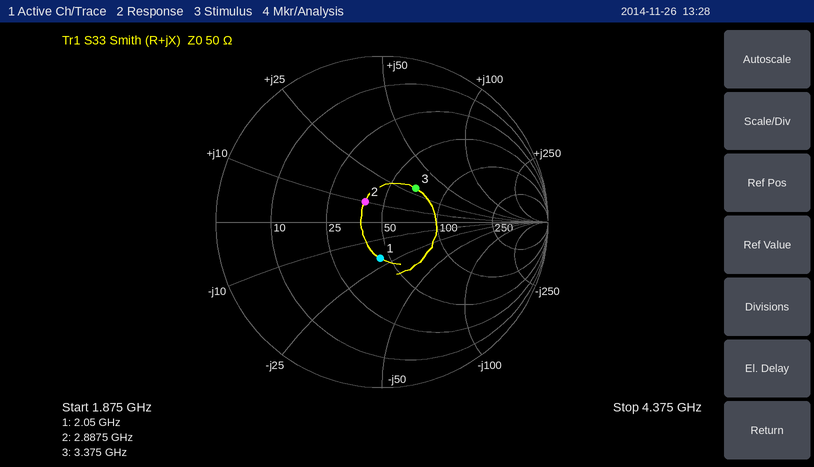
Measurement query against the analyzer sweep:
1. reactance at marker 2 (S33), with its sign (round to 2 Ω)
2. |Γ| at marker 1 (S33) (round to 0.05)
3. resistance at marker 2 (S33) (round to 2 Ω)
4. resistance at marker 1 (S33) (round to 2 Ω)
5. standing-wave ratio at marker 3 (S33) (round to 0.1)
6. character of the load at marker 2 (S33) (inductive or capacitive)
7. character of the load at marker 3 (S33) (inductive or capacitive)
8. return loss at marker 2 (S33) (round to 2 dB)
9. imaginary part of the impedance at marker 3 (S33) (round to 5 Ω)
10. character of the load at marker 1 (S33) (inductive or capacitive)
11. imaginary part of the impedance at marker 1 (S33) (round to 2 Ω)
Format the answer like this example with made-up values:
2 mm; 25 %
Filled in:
+10 Ω; 0.20; 40 Ω; 44 Ω; 1.8; inductive; inductive; 16 dB; +30 Ω; capacitive; -20 Ω
